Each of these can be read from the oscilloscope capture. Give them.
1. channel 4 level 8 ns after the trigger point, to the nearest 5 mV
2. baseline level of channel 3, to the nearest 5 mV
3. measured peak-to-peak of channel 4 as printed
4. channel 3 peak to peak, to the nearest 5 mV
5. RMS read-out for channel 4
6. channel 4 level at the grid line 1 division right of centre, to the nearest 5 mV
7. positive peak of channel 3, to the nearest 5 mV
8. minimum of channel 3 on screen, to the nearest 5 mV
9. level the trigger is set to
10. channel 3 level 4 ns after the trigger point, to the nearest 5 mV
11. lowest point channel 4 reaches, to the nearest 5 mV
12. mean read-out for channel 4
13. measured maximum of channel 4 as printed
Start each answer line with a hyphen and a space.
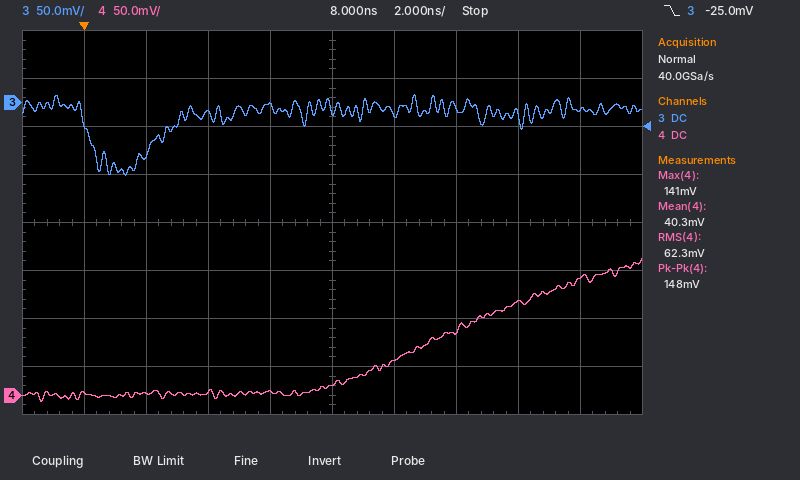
- 10 mV
- -10 mV
- 148 mV
- 85 mV
- 62.3 mV
- 35 mV
- 10 mV
- -75 mV
- -25.0 mV
- -10 mV
- -5 mV
- 40.3 mV
- 141 mV
